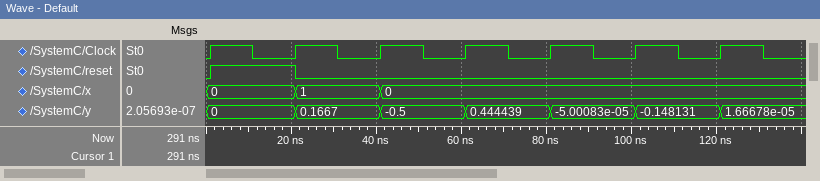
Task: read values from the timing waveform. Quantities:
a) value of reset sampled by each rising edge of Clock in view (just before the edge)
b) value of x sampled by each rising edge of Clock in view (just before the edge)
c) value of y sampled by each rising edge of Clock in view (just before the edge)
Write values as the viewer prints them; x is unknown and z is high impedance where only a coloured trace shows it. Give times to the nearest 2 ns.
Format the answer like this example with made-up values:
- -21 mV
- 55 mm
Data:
- 0 1 0 0 0 0 0
- 0, 0, 1, 0, 0, 0, 0
- 0, 0, 0.1667, -0.5, 0.444439, -5.00083e-05, -0.148131
